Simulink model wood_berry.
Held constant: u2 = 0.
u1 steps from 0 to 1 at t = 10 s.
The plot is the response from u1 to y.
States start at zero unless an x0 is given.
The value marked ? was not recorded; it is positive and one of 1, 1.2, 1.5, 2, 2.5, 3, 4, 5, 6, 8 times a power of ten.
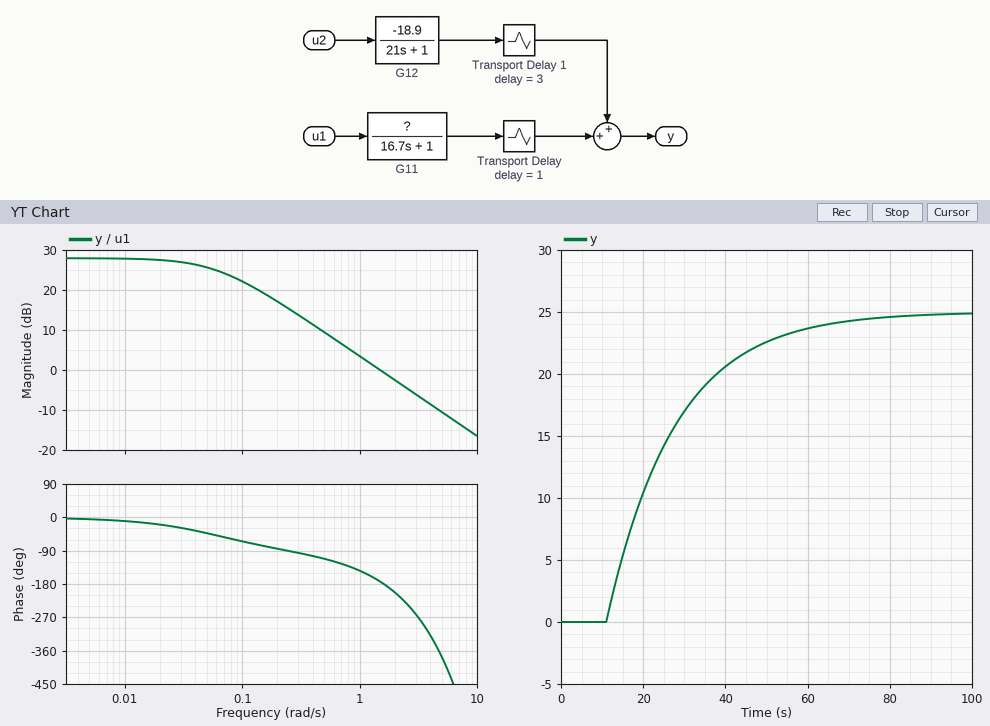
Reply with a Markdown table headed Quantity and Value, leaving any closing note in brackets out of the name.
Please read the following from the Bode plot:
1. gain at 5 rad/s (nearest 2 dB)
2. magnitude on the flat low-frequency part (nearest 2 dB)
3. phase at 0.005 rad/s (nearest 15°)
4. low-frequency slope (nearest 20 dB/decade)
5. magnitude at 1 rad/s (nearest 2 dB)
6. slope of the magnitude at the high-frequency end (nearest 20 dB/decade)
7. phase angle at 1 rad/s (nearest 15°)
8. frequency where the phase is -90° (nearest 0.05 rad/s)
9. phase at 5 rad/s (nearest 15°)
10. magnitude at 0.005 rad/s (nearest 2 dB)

| Quantity | Value |
|---|---|
| gain at 5 rad/s | -10 dB |
| magnitude on the flat low-frequency part | 28 dB |
| phase at 0.005 rad/s | 0° |
| low-frequency slope | 0 dB/decade |
| magnitude at 1 rad/s | 4 dB |
| slope of the magnitude at the high-frequency end | -20 dB/decade |
| phase angle at 1 rad/s | -150° |
| frequency where the phase is -90° | 0.25 rad/s |
| phase at 5 rad/s | -375° |
| magnitude at 0.005 rad/s | 28 dB |
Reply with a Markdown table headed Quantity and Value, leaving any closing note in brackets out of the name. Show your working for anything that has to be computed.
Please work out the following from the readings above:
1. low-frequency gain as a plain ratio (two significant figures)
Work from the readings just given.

| Quantity | Value |
|---|---|
| low-frequency gain as a plain ratio | 10^(28 / 20) = 25 |
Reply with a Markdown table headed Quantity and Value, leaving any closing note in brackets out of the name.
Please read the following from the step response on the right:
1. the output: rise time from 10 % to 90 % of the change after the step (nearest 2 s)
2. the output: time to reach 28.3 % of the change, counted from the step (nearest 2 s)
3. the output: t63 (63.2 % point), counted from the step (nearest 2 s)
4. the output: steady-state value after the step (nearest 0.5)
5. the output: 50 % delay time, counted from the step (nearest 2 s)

| Quantity | Value |
|---|---|
| the output: rise time from 10 % to 90 % of the change after the step | 36 s |
| the output: time to reach 28.3 % of the change, counted from the step | 6 s |
| the output: t63 (63.2 % point), counted from the step | 18 s |
| the output: steady-state value after the step | 25.0 |
| the output: 50 % delay time, counted from the step | 12 s |
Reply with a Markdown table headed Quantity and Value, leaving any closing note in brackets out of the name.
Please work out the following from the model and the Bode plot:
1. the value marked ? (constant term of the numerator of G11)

| Quantity | Value |
|---|---|
| the value marked ? | 25 |
